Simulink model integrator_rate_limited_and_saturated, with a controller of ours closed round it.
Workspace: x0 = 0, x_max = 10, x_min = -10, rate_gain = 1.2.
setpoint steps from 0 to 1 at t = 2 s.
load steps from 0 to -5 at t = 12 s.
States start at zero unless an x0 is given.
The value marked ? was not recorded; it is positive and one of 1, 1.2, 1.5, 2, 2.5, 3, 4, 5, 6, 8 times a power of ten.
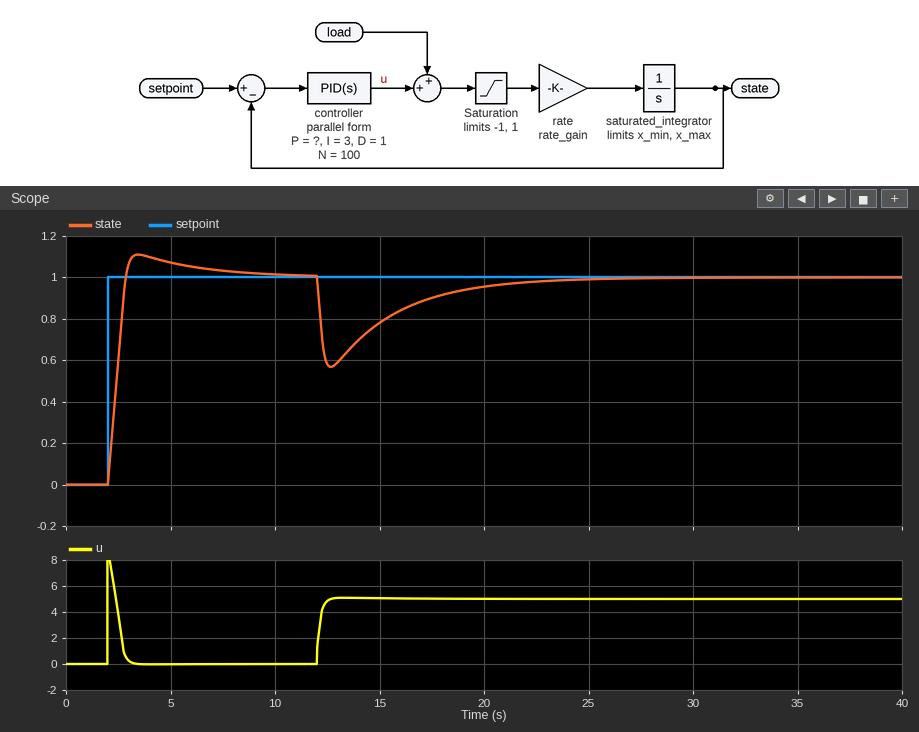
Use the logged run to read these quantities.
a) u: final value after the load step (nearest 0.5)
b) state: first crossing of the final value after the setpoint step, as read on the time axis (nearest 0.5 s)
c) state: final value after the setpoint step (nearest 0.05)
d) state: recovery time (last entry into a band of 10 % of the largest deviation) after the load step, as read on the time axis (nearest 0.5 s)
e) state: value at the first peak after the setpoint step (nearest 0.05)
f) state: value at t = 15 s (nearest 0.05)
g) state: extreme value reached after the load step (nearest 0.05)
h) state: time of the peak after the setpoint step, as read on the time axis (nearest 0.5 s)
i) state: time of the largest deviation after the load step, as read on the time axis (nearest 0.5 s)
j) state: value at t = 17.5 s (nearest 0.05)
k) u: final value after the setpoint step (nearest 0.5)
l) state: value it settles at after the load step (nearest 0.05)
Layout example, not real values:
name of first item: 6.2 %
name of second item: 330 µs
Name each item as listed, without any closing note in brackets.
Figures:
u: final value after the load step: 5.0
state: first crossing of the final value after the setpoint step, as read on the time axis: 3.0 s
state: final value after the setpoint step: 1.00
state: recovery time (last entry into a band of 10 % of the largest deviation) after the load step, as read on the time axis: 20.0 s
state: value at the first peak after the setpoint step: 1.10
state: value at t = 15 s: 0.80
state: extreme value reached after the load step: 0.55
state: time of the peak after the setpoint step, as read on the time axis: 3.5 s
state: time of the largest deviation after the load step, as read on the time axis: 12.5 s
state: value at t = 17.5 s: 0.90
u: final value after the setpoint step: 0.0
state: value it settles at after the load step: 1.00
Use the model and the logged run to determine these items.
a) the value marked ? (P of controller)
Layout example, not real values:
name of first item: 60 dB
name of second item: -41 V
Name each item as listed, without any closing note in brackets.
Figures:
the value marked ?: 10
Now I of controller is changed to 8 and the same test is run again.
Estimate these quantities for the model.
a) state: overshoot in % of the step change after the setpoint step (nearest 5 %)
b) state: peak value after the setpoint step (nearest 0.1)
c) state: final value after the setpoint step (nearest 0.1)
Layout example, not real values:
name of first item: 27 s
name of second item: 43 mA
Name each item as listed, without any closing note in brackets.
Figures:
state: overshoot in % of the step change after the setpoint step: 25 %
state: peak value after the setpoint step: 1.3
state: final value after the setpoint step: 1.0
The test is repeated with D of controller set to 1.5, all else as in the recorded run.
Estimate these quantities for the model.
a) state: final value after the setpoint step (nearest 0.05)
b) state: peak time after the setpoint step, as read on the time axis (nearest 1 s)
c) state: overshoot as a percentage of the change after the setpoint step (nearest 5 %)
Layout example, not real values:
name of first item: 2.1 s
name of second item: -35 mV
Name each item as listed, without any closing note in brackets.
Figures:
state: final value after the setpoint step: 1.00
state: peak time after the setpoint step, as read on the time axis: 4 s
state: overshoot as a percentage of the change after the setpoint step: 10 %
